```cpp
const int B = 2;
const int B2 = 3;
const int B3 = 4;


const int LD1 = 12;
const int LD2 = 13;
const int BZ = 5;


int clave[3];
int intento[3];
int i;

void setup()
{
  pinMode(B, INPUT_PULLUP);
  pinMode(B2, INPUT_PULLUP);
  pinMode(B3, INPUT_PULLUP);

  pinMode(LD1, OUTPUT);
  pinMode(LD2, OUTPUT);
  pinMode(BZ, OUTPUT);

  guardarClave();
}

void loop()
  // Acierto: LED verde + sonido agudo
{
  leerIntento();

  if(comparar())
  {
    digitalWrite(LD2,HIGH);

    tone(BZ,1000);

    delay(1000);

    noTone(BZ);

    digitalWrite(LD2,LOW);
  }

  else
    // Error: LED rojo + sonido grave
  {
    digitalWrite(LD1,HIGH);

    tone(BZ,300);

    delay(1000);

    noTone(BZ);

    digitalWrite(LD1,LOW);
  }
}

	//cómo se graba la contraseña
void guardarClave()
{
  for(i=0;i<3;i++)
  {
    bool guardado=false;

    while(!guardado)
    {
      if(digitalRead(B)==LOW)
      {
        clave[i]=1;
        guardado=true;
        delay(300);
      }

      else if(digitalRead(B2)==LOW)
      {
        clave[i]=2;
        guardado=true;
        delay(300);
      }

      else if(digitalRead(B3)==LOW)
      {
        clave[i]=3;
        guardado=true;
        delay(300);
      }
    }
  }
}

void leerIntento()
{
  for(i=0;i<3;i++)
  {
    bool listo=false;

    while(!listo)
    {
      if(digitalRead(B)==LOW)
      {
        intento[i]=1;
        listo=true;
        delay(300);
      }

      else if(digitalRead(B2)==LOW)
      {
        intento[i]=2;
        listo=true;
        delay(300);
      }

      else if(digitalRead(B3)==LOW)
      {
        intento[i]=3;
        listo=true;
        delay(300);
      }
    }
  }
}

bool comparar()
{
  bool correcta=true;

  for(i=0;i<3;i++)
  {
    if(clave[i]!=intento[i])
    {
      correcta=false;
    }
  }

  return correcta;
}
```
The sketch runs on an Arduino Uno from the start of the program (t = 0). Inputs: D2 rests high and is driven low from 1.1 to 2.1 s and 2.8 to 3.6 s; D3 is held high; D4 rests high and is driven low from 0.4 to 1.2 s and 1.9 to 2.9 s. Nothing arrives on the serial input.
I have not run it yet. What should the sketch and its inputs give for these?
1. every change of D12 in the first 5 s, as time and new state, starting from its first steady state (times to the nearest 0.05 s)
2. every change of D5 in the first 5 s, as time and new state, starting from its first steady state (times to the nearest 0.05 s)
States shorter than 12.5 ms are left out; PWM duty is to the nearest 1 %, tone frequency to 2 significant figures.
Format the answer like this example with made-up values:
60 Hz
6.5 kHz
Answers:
0 s low; 2.2 s high; 3.2 s low
0 s low; 2.2 s tone 300 Hz; 3.2 s low
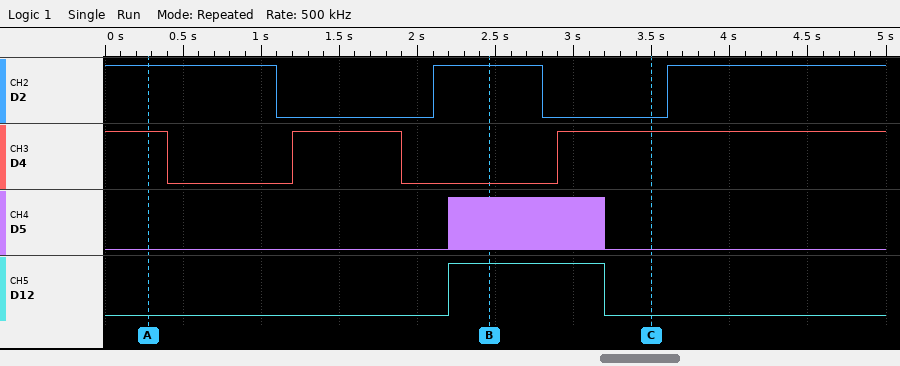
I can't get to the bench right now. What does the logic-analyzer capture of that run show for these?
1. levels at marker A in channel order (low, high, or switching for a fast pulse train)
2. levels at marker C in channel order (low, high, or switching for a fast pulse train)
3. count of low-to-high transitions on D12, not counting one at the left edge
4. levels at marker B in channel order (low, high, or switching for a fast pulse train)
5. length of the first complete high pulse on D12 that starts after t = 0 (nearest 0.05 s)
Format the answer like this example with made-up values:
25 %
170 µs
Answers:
D2 high, D4 high, D5 low, D12 low
D2 low, D4 high, D5 low, D12 low
1
D2 high, D4 low, D5 switching, D12 high
1.00 s
